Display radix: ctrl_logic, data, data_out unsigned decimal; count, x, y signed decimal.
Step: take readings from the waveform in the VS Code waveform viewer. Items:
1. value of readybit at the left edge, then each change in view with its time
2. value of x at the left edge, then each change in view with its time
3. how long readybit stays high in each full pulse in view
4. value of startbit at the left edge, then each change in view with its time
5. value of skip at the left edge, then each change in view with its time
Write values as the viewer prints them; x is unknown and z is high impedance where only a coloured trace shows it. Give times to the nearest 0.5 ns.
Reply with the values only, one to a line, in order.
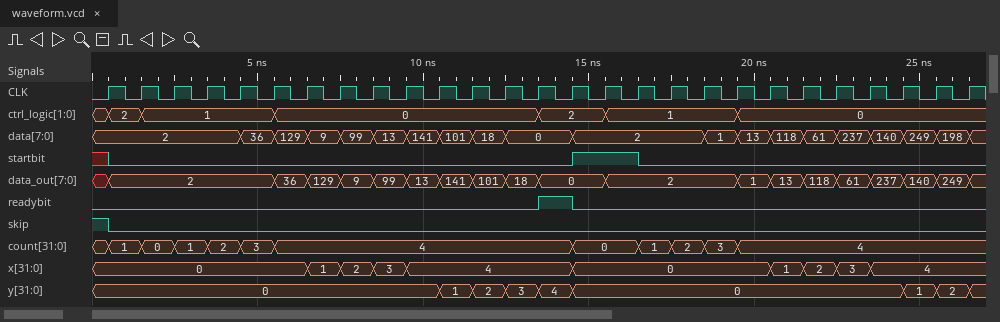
0, 1 at 13.5 ns, 0 at 14.5 ns
0, 1 at 6.5 ns, 2 at 7.5 ns, 3 at 8.5 ns, 4 at 9.5 ns, 0 at 14.5 ns, 1 at 20.5 ns, 2 at 21.5 ns, 3 at 22.5 ns, 4 at 23.5 ns
1 ns
x, 0 at 0.5 ns, 1 at 14.5 ns, 0 at 16.5 ns
1, 0 at 0.5 ns
